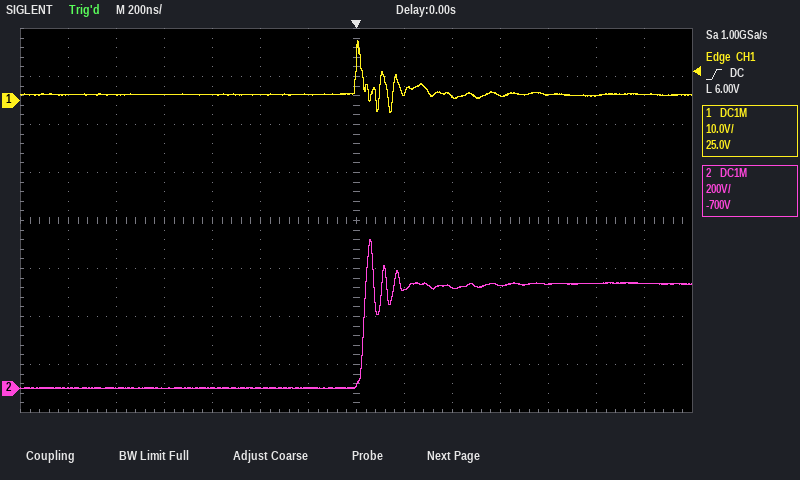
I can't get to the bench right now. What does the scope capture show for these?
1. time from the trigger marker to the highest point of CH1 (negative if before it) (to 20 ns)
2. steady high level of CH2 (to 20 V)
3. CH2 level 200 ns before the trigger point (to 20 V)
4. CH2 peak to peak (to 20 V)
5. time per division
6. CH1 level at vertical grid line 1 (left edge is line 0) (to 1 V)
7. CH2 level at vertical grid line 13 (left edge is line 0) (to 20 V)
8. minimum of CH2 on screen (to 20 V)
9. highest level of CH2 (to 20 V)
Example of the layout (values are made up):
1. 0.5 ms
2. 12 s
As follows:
1. 0 ns
2. 440 V
3. 0 V
4. 620 V
5. 200 ns
6. 1 V
7. 440 V
8. 0 V
9. 620 V
